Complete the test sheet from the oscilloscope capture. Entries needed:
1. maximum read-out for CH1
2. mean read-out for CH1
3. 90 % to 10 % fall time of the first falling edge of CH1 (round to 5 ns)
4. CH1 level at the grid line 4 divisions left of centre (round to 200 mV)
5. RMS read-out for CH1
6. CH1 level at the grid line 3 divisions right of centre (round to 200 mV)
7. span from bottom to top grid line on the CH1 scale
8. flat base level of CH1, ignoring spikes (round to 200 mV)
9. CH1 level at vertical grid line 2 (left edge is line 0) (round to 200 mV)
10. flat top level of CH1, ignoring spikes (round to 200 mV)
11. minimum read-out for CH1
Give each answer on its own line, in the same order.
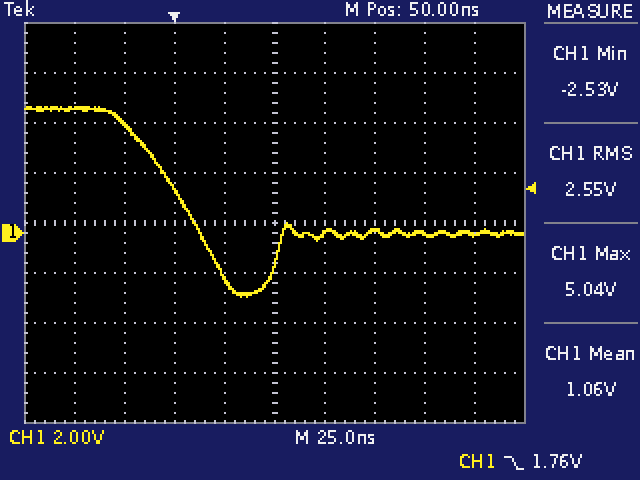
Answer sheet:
5.04 V
1.06 V
35 ns
5.0 V
2.55 V
0.0 V
16 V
0.0 V
4.4 V
5.0 V
-2.53 V
